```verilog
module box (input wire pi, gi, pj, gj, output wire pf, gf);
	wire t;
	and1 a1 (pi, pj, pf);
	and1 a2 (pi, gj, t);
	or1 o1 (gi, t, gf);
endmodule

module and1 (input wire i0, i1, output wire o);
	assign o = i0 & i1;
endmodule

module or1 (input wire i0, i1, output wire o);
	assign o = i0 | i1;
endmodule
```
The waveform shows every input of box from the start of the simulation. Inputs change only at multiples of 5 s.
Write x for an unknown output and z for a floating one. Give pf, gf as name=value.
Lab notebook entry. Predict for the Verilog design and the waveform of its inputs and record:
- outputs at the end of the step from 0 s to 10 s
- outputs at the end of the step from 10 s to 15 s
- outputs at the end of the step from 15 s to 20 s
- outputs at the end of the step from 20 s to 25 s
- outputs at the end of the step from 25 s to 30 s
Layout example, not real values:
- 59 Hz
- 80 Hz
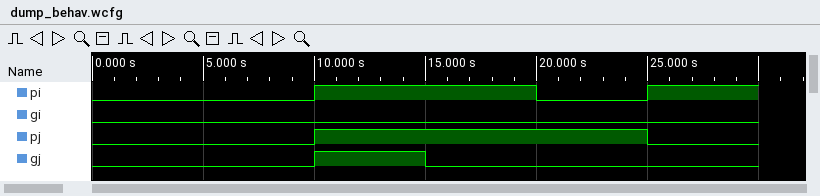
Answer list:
- pf=0, gf=0
- pf=1, gf=1
- pf=1, gf=0
- pf=0, gf=0
- pf=0, gf=0
